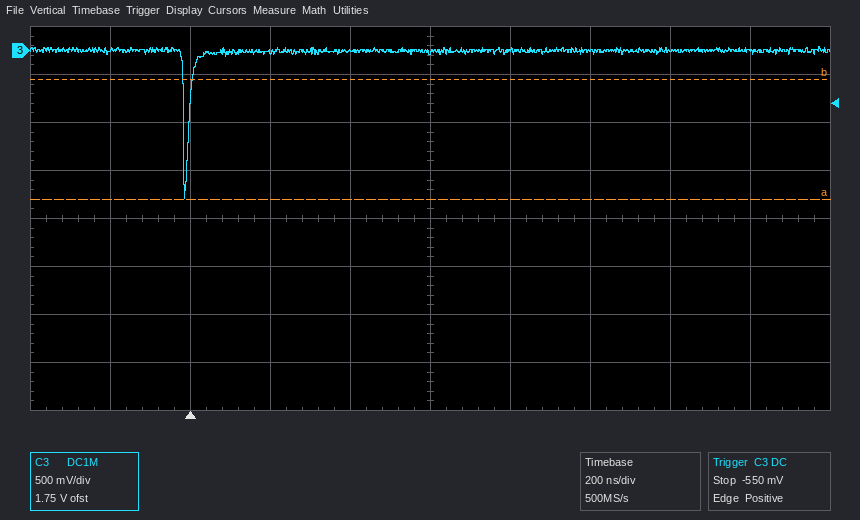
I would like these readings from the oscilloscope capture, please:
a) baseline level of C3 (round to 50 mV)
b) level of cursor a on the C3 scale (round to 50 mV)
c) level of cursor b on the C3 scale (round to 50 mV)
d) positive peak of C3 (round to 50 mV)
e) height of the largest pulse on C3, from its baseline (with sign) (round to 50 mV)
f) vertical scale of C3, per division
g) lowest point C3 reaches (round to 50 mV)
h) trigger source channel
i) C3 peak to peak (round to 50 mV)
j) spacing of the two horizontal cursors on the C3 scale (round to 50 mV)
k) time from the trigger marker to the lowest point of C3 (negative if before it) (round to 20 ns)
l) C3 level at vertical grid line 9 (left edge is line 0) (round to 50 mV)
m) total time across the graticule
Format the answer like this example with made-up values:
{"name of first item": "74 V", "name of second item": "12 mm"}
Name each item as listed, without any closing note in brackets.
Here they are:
{"baseline level of C3": "0 mV", "level of cursor a on the C3 scale": "-1.55 V", "level of cursor b on the C3 scale": "-300 mV", "positive peak of C3": "50 mV", "height of the largest pulse on C3, from its baseline (with sign)": "-1.55 V", "vertical scale of C3, per division": "500 mV", "lowest point C3 reaches": "-1.55 V", "trigger source channel": "C3", "C3 peak to peak": "1.60 V", "spacing of the two horizontal cursors on the C3 scale": "1.25 V", "time from the trigger marker to the lowest point of C3 (negative if before it)": "-20 ns", "C3 level at vertical grid line 9 (left edge is line 0)": "0 mV", "total time across the graticule": "2 µs"}
